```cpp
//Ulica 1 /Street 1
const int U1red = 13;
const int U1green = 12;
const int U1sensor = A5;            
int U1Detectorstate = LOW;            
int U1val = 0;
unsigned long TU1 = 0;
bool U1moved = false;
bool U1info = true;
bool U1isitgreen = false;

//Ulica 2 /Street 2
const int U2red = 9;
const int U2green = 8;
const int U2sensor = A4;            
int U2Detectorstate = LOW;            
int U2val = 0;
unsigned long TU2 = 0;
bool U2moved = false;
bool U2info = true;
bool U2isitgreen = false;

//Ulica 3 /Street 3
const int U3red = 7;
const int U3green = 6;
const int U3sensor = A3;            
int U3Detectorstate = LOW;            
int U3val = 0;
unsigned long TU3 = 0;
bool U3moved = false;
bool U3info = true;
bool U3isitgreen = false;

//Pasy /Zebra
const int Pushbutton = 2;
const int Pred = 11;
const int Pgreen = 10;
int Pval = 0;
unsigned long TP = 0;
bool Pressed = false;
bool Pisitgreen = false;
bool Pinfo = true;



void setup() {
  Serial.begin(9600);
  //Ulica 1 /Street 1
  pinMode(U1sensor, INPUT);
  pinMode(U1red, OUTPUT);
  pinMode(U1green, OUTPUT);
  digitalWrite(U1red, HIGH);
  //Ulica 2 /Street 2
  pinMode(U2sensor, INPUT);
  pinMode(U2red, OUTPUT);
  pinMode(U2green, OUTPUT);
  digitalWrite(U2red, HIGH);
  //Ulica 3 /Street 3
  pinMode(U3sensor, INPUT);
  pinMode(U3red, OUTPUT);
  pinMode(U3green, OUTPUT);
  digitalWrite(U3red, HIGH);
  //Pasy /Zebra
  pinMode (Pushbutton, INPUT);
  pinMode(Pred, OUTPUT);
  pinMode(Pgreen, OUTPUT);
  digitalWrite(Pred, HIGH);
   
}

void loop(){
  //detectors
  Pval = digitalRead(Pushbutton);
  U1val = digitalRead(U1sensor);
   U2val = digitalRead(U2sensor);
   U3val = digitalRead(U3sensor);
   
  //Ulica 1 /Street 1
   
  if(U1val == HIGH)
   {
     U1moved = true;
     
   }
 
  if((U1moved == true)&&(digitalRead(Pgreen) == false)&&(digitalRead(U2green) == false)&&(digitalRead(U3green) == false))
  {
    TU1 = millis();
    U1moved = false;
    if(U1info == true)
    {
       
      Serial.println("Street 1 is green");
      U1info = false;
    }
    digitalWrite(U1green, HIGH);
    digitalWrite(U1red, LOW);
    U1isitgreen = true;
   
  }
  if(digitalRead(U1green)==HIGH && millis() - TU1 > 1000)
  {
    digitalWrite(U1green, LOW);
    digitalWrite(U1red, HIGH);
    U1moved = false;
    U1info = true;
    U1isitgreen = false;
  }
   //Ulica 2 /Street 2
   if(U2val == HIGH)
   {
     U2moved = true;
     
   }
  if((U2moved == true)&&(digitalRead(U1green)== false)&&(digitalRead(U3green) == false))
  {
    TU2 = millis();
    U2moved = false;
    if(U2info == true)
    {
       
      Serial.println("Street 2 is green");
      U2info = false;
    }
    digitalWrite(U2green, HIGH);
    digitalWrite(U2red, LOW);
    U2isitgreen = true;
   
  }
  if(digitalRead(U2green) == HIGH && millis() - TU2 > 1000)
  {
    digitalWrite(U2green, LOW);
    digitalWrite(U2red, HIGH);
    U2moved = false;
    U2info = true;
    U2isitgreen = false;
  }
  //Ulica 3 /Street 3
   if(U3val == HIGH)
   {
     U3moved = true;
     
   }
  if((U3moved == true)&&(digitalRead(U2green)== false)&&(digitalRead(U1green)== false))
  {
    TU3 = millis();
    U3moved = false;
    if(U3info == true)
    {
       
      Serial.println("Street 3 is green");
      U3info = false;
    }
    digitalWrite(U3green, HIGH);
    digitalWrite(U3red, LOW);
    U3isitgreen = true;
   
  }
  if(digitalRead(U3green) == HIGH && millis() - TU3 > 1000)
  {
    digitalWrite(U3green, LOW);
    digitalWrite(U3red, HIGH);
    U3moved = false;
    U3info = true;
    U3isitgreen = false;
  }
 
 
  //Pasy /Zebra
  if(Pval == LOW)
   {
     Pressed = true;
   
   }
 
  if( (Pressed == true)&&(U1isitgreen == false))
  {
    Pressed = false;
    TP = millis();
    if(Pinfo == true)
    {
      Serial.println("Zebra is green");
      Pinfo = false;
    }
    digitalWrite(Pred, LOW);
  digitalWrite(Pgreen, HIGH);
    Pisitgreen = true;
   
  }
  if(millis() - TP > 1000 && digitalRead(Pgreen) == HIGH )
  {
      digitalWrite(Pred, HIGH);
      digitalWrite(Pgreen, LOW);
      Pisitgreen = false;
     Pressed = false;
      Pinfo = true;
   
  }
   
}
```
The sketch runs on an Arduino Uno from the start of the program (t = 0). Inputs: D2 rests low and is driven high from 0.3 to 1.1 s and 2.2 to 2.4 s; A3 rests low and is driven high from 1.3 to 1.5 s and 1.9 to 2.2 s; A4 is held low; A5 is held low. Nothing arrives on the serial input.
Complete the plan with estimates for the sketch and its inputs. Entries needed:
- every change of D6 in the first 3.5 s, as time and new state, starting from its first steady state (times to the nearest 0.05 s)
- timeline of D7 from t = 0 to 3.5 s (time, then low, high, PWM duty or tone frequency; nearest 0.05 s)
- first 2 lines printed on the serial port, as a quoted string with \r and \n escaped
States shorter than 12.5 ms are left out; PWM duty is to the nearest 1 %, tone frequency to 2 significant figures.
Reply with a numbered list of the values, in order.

1. 0 s low; 1.3 s high; 3.2 s low
2. 0 s high; 1.3 s low; 3.2 s high
3. "Zebra is green\r\nStreet 3 is green\r\n"
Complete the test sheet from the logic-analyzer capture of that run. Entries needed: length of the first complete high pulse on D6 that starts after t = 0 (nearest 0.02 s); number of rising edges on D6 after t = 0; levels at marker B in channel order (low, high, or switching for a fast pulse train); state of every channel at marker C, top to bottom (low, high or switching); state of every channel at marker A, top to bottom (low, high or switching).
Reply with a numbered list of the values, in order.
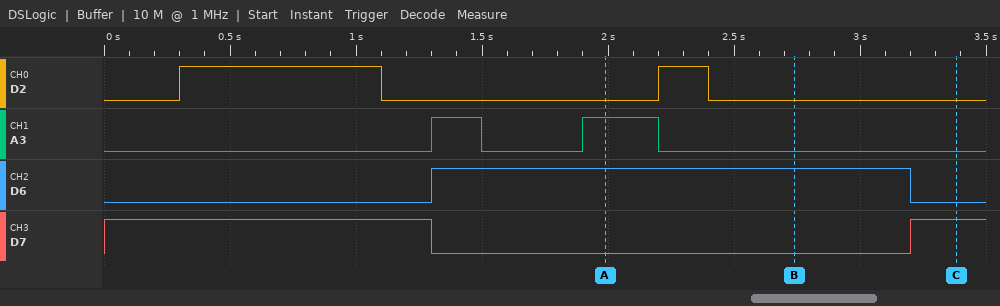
1. 1.90 s
2. 1
3. D2 low, A3 low, D6 high, D7 low
4. D2 low, A3 low, D6 low, D7 high
5. D2 low, A3 high, D6 high, D7 low
